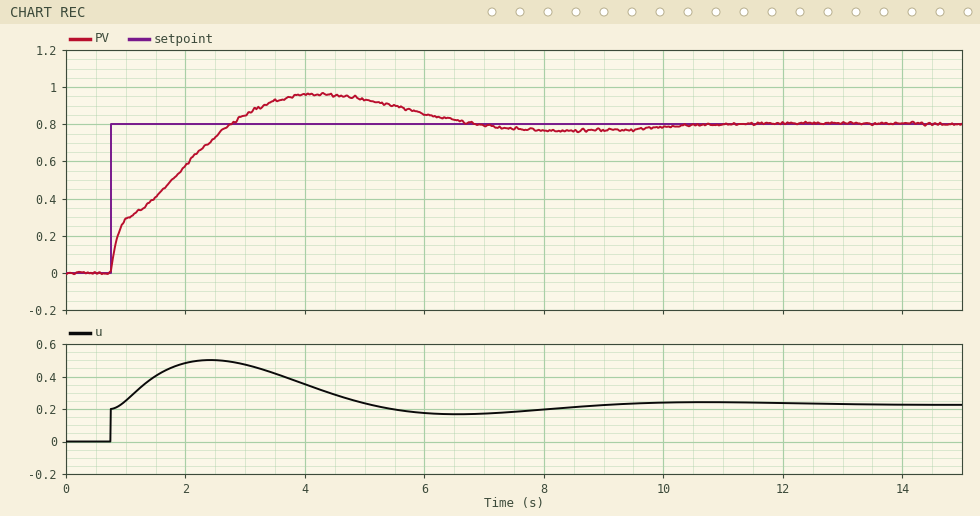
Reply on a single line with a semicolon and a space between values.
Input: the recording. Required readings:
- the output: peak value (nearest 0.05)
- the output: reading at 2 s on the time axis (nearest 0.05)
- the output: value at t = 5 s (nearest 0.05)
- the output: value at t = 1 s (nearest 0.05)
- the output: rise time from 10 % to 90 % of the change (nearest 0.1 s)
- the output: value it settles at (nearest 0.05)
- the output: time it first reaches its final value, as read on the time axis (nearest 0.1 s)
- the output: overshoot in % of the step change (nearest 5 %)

0.95; 0.60; 0.95; 0.30; 1.7 s; 0.80; 2.8 s; 20 %
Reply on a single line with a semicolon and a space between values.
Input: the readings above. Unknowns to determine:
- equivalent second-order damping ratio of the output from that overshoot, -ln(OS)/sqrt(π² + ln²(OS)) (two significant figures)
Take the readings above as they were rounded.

0.46
